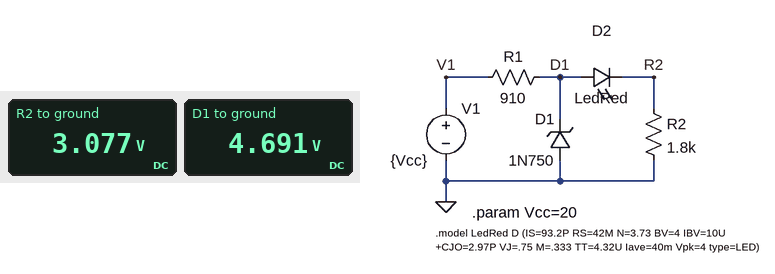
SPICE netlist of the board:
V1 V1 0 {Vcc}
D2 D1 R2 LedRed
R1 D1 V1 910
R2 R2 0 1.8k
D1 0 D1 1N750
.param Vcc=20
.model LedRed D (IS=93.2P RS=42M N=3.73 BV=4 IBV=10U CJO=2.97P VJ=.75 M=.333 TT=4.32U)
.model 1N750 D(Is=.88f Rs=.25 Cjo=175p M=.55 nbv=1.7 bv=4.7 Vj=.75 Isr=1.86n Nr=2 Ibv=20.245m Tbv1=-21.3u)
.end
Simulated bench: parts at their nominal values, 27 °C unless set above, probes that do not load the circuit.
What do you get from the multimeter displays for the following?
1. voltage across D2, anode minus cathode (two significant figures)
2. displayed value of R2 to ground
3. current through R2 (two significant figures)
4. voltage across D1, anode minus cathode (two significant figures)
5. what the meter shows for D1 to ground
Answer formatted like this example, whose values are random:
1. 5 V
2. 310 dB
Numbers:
1. 1.6 V
2. 3.077 V
3. 1.7 mA
4. -4.7 V
5. 4.691 V
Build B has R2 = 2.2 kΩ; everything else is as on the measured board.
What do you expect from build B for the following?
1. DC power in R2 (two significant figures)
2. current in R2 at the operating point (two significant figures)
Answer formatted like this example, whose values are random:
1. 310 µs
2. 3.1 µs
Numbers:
1. 4.4 mW
2. 1.4 mA
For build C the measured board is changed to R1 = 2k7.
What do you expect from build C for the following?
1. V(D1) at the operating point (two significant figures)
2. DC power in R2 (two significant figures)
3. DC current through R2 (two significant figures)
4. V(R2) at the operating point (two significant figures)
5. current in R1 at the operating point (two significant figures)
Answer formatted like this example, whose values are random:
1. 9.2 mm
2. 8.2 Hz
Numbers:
1. 4.6 V
2. 5.1 mW
3. 1.7 mA
4. 3.0 V
5. 5.7 mA
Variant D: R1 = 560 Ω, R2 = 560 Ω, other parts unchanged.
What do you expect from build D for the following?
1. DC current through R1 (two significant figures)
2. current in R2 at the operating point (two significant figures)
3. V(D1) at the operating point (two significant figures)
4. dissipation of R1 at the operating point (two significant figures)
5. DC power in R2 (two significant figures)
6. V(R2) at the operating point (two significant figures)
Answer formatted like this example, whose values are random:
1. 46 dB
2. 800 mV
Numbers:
1. 27 mA
2. 5.3 mA
3. 4.7 V
4. 420 mW
5. 16 mW
6. 3.0 V
